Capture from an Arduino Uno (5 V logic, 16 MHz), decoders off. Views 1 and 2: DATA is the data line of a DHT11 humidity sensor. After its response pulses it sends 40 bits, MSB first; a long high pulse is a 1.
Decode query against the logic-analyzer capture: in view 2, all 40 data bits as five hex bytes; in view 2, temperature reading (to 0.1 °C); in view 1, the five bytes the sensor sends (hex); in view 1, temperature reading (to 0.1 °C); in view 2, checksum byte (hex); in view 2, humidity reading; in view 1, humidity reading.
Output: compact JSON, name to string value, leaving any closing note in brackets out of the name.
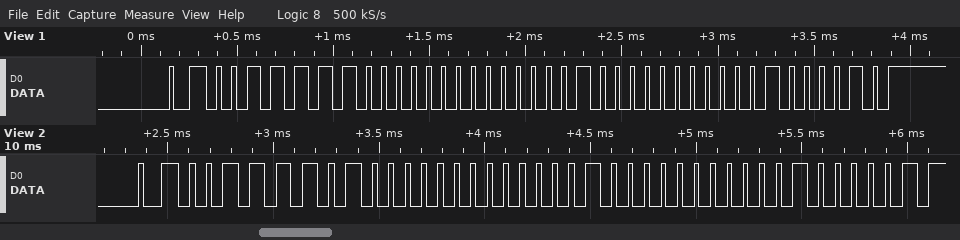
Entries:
{"in view 2, all 40 data bits as five hex bytes": "3D 00 04 00 41", "in view 2, temperature reading": "4.0 °C", "in view 1, the five bytes the sensor sends": "3E 00 04 00 42", "in view 1, temperature reading": "4.0 °C", "in view 2, checksum byte": "0x41", "in view 2, humidity reading": "61 %", "in view 1, humidity reading": "62 %"}
